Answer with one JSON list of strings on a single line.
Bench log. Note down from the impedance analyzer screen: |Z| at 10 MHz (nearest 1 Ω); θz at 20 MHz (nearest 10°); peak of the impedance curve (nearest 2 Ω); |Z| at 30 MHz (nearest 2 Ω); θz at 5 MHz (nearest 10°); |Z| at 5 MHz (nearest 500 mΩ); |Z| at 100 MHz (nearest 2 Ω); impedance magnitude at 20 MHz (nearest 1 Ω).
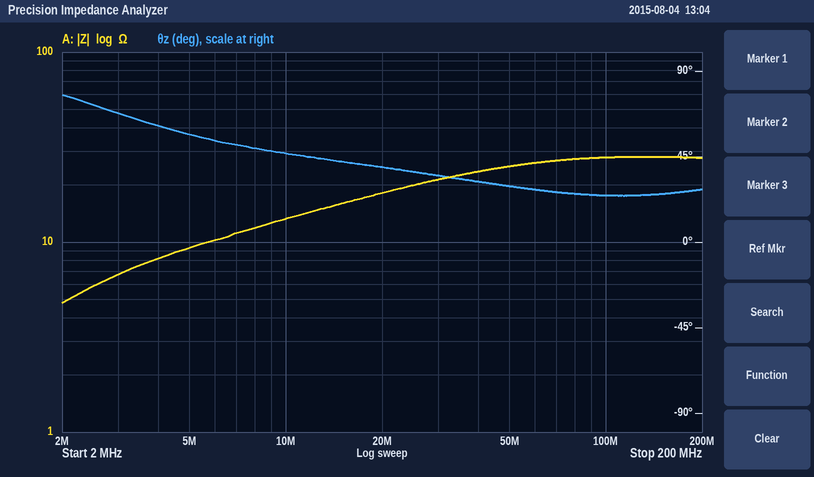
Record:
["13 Ω", "40°", "28 Ω", "22 Ω", "60°", "9.5 Ω", "28 Ω", "18 Ω"]
